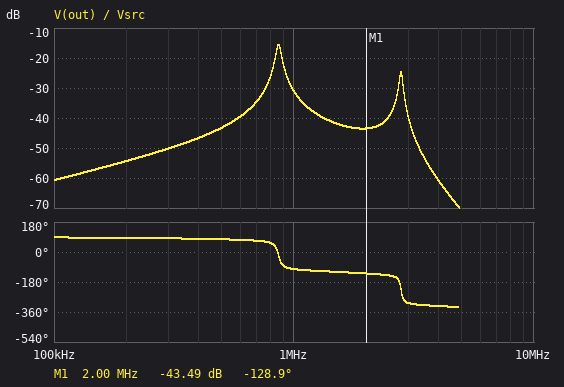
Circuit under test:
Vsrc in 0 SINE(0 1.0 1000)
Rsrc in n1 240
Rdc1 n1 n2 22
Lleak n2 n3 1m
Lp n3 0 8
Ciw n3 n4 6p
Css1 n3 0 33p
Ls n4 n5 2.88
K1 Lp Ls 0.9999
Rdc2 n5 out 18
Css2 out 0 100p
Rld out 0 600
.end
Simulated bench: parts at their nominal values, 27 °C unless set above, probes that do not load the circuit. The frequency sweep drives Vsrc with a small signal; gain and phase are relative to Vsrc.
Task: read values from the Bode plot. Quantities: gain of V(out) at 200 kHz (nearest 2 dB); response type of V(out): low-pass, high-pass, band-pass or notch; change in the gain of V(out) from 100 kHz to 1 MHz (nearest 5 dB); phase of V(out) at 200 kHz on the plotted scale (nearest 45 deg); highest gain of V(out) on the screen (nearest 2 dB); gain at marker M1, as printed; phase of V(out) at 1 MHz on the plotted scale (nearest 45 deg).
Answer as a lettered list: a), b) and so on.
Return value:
a) -54 dB
b) band-pass
c) 30 dB
d) 90 deg
e) -16 dB
f) -43.49 dB
g) -90 deg
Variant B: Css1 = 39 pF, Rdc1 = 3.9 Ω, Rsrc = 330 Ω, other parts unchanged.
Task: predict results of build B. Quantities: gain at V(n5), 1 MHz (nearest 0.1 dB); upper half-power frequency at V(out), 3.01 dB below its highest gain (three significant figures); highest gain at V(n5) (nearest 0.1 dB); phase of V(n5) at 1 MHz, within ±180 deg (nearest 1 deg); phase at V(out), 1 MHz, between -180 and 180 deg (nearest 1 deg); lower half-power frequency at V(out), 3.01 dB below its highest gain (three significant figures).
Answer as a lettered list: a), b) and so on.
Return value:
a) -35.4 dB
b) 823 kHz
c) -18.8 dB
d) -103 deg
e) -104 deg
f) 769 kHz
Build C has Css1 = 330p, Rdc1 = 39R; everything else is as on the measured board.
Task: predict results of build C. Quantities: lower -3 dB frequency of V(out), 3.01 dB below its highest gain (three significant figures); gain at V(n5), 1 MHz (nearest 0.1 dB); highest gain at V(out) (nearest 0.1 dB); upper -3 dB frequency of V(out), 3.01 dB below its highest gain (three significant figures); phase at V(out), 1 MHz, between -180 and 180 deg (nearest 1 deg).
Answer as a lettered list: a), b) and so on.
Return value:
a) 255 kHz
b) -61.6 dB
c) -36.1 dB
d) 300 kHz
e) -109 deg
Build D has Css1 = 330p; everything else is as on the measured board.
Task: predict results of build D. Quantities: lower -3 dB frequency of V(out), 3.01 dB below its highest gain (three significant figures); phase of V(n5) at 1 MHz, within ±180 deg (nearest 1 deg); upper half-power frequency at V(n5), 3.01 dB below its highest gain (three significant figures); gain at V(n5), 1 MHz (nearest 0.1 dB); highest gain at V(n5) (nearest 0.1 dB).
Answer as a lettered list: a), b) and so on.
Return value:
a) 257 kHz
b) -109 deg
c) 298 kHz
d) -61.6 dB
e) -35.3 dB
